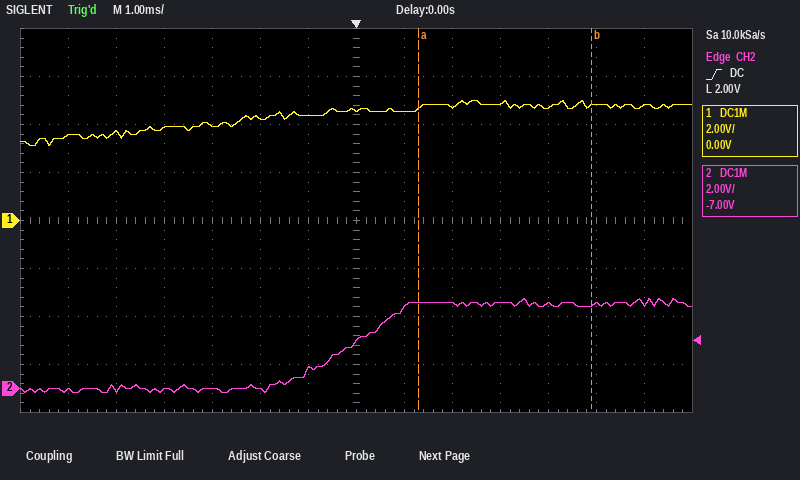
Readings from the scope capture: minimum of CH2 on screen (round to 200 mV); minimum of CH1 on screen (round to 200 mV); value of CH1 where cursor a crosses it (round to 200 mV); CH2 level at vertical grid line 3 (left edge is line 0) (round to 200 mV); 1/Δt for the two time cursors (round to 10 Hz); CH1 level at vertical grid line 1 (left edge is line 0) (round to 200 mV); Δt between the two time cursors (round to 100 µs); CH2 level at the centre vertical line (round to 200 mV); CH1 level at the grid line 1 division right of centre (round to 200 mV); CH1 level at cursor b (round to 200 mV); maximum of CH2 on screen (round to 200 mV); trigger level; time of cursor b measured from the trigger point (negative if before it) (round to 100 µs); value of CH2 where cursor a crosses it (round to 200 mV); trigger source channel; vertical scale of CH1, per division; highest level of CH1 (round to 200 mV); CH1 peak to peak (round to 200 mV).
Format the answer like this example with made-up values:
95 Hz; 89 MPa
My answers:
-200 mV; 3.2 V; 4.6 V; 0.0 V; 280 Hz; 3.6 V; 3.6 ms; 2.0 V; 4.6 V; 4.8 V; 3.8 V; 2.00 V; +4.9 ms; 3.6 V; CH2; 2 V; 5.0 V; 1.8 V
